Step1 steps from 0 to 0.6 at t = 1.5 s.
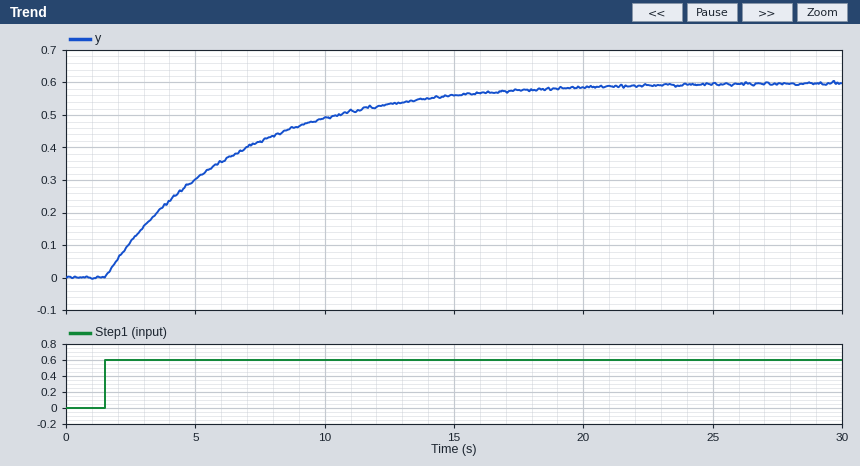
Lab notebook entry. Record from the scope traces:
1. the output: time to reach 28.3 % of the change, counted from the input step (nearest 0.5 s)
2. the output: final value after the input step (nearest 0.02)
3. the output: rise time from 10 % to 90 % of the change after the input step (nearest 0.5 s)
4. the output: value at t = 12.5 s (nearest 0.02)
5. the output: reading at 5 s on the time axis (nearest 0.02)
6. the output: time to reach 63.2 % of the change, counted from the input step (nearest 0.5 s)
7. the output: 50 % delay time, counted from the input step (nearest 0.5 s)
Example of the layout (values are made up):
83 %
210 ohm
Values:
1.5 s
0.60
11.0 s
0.54
0.30
5.0 s
3.5 s
